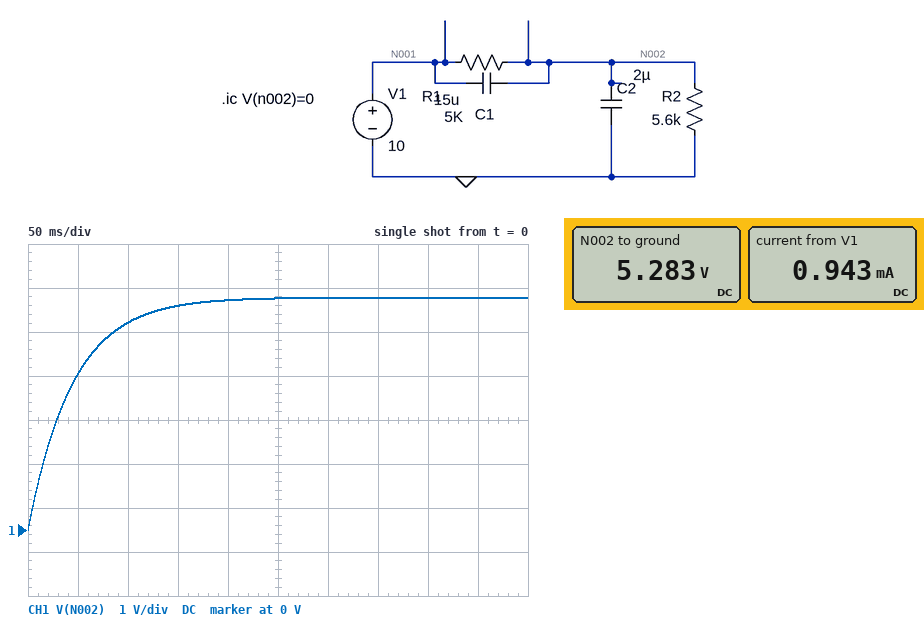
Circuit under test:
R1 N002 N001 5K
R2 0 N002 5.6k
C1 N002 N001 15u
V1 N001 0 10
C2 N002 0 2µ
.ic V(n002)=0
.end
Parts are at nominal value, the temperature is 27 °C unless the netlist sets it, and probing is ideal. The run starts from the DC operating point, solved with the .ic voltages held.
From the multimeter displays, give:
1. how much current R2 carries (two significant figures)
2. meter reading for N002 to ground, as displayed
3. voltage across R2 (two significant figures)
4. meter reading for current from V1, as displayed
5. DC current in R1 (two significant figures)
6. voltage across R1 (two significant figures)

940 µA
5.283 V
5.3 V
0.943 mA
940 µA
4.7 V
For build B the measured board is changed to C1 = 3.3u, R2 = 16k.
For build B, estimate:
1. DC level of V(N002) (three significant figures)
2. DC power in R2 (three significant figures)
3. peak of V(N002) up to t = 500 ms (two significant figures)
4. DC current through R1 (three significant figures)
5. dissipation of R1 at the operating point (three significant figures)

7.62 V
3.63 mW
7.6 V
476 µA
1.13 mW
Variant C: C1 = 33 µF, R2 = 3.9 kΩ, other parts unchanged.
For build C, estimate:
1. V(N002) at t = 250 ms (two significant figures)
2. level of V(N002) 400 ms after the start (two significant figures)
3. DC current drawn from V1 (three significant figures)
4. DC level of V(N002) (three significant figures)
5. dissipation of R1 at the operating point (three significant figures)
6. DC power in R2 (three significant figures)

4.2 V
4.4 V
1.12 mA
4.38 V
6.31 mW
4.92 mW
